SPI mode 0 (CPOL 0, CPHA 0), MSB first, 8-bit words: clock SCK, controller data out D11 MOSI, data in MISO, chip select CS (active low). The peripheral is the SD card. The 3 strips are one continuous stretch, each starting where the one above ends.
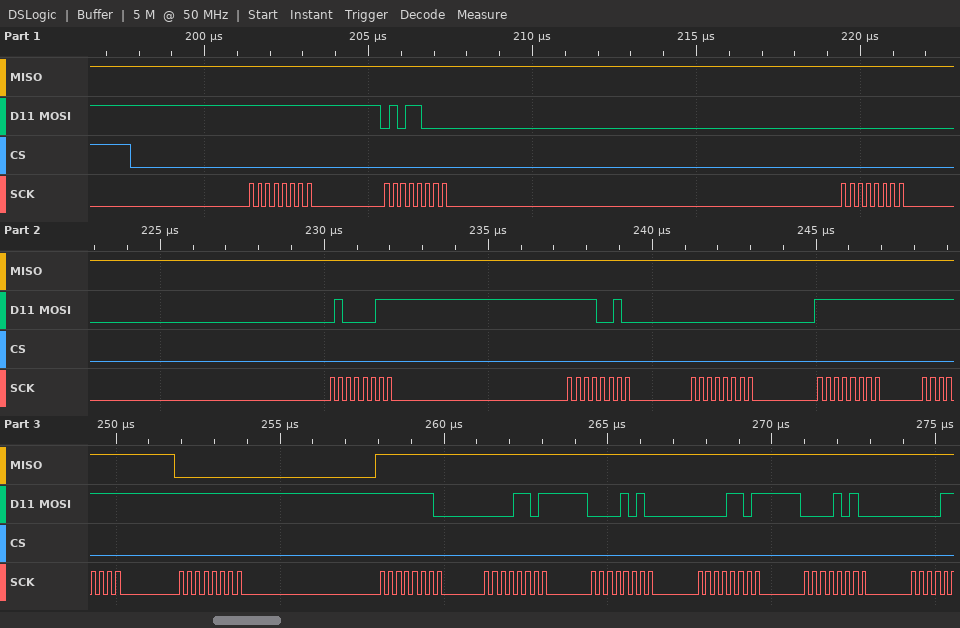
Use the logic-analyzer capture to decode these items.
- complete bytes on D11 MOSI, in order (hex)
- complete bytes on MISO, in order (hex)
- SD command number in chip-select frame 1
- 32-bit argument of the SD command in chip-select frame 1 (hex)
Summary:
FF 58 00 43 F2 00 FF FF FF FE 0D 0A 0D 0A
FF FF FF FF FF FF FF FF 00 FF FF FF FF FF
CMD24
0x0043F200
